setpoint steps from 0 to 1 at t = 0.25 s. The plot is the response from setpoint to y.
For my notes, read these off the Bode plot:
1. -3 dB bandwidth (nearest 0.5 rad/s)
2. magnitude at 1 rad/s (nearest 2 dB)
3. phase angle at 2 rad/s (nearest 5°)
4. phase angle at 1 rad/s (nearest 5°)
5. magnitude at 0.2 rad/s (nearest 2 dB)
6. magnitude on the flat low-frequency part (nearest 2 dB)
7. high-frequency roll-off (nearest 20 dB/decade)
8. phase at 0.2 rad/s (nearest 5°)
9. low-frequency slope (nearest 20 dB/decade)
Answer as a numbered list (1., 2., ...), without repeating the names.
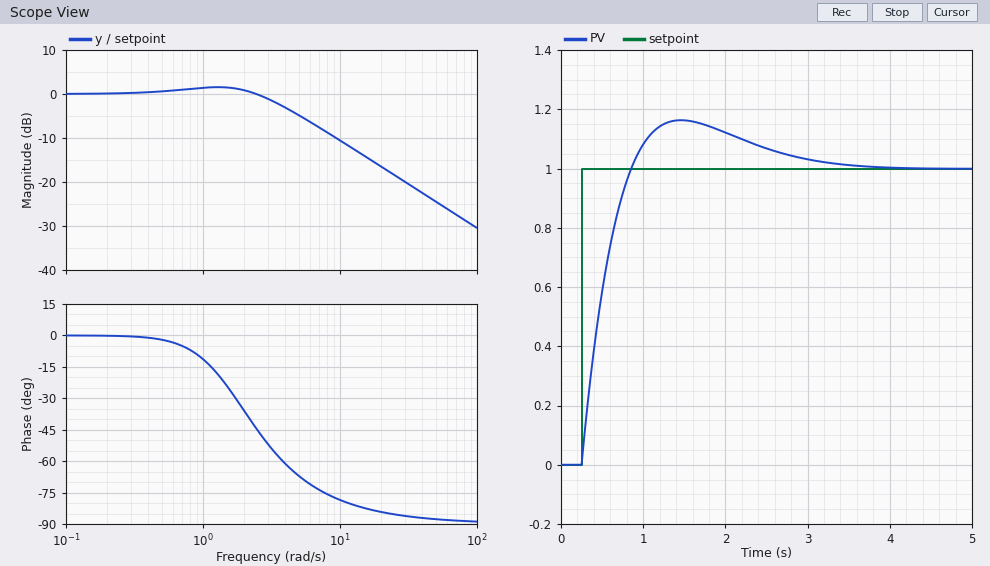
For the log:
1. 4.0 rad/s
2. 2 dB
3. -35°
4. -10°
5. 0 dB
6. 0 dB
7. -20 dB/decade
8. 0°
9. 0 dB/decade
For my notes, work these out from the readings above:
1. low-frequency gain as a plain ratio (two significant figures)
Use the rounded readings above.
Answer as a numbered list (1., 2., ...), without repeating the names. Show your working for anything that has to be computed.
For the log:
1. 10^(0 / 20) = 1.0
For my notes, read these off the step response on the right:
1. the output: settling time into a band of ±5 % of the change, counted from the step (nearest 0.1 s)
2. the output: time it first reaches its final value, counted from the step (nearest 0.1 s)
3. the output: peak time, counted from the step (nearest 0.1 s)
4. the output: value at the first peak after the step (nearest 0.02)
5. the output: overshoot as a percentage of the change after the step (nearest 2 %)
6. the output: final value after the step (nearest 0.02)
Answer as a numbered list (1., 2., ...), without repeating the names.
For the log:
1. 2.5 s
2. 0.6 s
3. 1.2 s
4. 1.16
5. 16 %
6. 1.00
